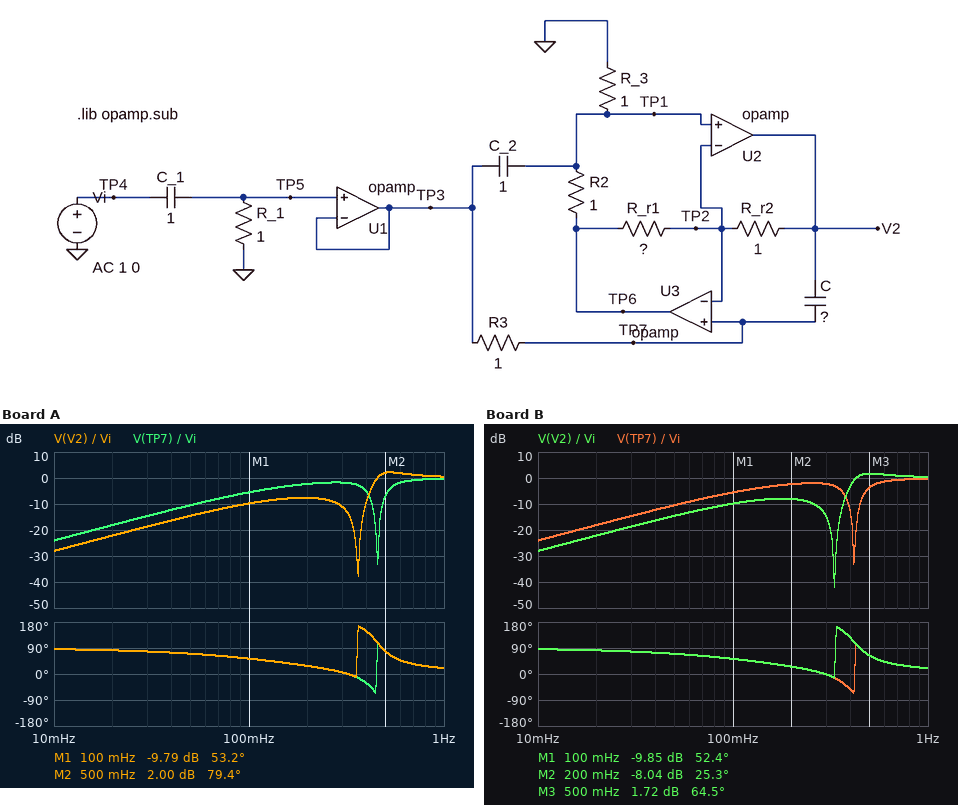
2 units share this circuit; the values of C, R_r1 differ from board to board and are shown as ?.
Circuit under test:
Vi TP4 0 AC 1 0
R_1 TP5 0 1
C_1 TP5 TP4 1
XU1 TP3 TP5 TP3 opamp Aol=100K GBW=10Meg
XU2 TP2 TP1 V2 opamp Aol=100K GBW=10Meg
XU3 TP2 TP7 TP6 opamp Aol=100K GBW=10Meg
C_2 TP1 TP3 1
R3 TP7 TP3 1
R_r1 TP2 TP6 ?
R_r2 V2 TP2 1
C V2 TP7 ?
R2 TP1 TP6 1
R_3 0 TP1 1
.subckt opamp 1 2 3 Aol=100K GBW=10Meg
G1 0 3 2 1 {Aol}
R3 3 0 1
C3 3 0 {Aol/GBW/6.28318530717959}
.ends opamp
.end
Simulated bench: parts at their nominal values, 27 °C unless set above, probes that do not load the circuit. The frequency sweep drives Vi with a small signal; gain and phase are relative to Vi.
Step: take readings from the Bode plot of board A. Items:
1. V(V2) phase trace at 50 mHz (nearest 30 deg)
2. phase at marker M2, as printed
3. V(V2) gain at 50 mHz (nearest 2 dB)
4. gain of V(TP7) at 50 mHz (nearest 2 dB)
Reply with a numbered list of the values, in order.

1. 60 deg
2. 79.4 deg
3. -14 dB
4. -10 dB
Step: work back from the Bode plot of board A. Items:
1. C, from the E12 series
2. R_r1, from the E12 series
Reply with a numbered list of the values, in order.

1. 330 mF
2. 2.7 Ω
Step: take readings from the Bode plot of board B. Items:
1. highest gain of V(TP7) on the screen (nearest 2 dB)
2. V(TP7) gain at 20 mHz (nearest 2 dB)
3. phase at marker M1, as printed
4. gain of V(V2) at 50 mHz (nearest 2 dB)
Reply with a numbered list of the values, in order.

1. 0 dB
2. -18 dB
3. 52.4 deg
4. -14 dB
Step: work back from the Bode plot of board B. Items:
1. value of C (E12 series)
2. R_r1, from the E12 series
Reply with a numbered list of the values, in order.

1. 390 mF
2. 2.7 Ω
